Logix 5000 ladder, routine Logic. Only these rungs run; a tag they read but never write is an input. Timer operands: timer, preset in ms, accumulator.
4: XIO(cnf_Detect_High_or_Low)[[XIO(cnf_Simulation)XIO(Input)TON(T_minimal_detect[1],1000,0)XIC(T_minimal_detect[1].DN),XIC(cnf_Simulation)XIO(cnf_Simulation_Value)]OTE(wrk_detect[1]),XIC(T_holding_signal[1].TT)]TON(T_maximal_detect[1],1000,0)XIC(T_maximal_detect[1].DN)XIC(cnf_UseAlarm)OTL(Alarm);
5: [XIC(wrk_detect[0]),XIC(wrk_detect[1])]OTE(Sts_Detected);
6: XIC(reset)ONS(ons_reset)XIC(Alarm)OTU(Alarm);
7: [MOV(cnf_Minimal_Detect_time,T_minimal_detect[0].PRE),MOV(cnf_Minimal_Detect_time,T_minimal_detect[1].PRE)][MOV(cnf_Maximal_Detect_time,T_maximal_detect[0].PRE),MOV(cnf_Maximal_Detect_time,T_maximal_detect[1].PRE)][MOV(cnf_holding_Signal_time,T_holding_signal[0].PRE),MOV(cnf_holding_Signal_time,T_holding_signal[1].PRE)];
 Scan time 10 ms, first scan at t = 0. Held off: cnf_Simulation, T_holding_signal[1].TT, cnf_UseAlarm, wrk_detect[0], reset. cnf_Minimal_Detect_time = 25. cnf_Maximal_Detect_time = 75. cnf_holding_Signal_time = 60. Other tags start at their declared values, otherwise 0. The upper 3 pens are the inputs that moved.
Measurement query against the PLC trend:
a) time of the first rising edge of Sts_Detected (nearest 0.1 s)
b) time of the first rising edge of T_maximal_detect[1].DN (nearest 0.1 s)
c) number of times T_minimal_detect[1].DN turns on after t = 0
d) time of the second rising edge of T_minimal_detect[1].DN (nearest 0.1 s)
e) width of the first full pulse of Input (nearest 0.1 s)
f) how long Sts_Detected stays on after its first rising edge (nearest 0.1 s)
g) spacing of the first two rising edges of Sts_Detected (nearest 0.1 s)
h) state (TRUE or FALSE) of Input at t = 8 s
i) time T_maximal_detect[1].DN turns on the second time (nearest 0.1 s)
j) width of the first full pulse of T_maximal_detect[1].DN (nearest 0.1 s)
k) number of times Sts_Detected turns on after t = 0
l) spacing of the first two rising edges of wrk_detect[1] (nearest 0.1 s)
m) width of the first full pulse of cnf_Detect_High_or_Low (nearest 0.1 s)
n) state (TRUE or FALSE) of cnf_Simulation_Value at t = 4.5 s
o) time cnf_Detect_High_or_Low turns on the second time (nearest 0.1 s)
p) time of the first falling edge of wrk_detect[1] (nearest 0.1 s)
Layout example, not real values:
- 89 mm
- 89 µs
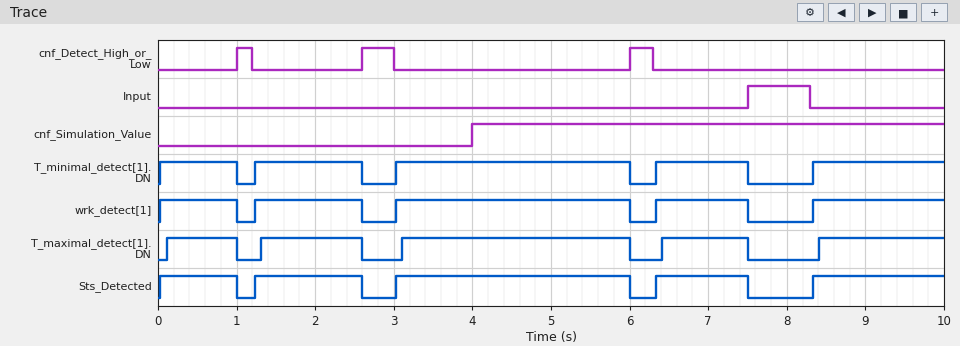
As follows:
- 0.0 s
- 0.1 s
- 5
- 1.2 s
- 0.8 s
- 1.0 s
- 1.2 s
- TRUE
- 1.3 s
- 0.9 s
- 5
- 1.2 s
- 0.2 s
- TRUE
- 2.6 s
- 1.0 s
